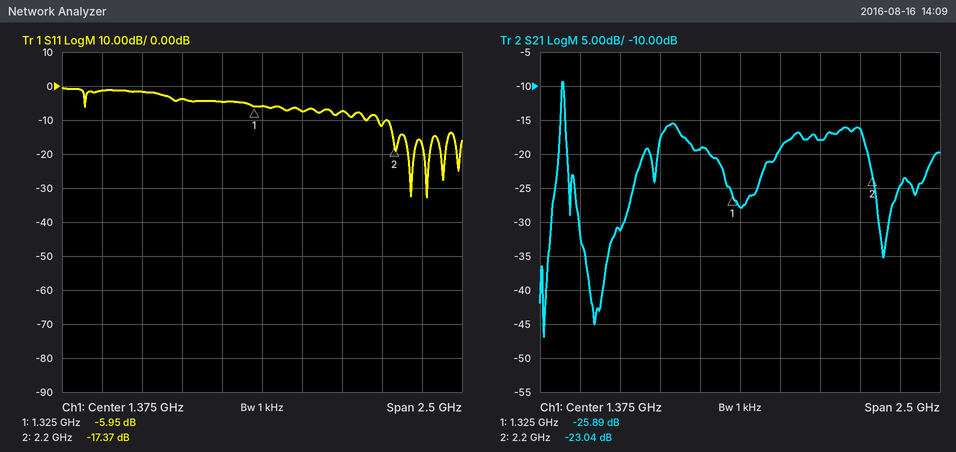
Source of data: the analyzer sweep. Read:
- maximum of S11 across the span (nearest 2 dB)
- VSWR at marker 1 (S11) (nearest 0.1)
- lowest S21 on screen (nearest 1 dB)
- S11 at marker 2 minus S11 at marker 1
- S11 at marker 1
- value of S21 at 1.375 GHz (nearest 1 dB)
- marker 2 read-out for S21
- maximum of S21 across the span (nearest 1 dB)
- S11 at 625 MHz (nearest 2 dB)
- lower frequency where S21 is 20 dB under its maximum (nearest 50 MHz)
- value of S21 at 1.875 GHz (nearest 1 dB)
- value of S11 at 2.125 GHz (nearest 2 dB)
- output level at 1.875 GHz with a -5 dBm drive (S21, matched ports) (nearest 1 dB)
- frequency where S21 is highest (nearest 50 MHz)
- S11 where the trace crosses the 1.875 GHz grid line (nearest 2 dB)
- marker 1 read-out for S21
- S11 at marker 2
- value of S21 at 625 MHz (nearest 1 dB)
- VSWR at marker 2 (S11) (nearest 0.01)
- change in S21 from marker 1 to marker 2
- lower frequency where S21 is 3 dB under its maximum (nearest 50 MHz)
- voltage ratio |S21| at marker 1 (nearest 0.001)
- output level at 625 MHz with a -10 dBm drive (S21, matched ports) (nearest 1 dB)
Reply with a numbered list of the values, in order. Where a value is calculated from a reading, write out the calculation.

1. 0 dB
2. (1 + 0.5041)/(1 − 0.5041) ≈ 3.0
3. -47 dB
4. -17.37 − (-5.95) = -11.42 dB
5. -5.95 dB
6. -28 dB
7. -23.04 dB
8. -9 dB
9. -2 dB
10. 200 MHz
11. -18 dB
12. -12 dB
13. -5 dBm + (-18 dB) = -23 dBm
14. 250 MHz
15. -8 dB
16. -25.89 dB
17. -17.37 dB
18. -31 dB
19. (1 + 0.1354)/(1 − 0.1354) ≈ 1.31
20. -23.04 − (-25.89) = 2.85 dB
21. 250 MHz
22. 10^(-25.89/20) ≈ 0.051
23. -10 dBm + (-31 dB) = -41 dBm
